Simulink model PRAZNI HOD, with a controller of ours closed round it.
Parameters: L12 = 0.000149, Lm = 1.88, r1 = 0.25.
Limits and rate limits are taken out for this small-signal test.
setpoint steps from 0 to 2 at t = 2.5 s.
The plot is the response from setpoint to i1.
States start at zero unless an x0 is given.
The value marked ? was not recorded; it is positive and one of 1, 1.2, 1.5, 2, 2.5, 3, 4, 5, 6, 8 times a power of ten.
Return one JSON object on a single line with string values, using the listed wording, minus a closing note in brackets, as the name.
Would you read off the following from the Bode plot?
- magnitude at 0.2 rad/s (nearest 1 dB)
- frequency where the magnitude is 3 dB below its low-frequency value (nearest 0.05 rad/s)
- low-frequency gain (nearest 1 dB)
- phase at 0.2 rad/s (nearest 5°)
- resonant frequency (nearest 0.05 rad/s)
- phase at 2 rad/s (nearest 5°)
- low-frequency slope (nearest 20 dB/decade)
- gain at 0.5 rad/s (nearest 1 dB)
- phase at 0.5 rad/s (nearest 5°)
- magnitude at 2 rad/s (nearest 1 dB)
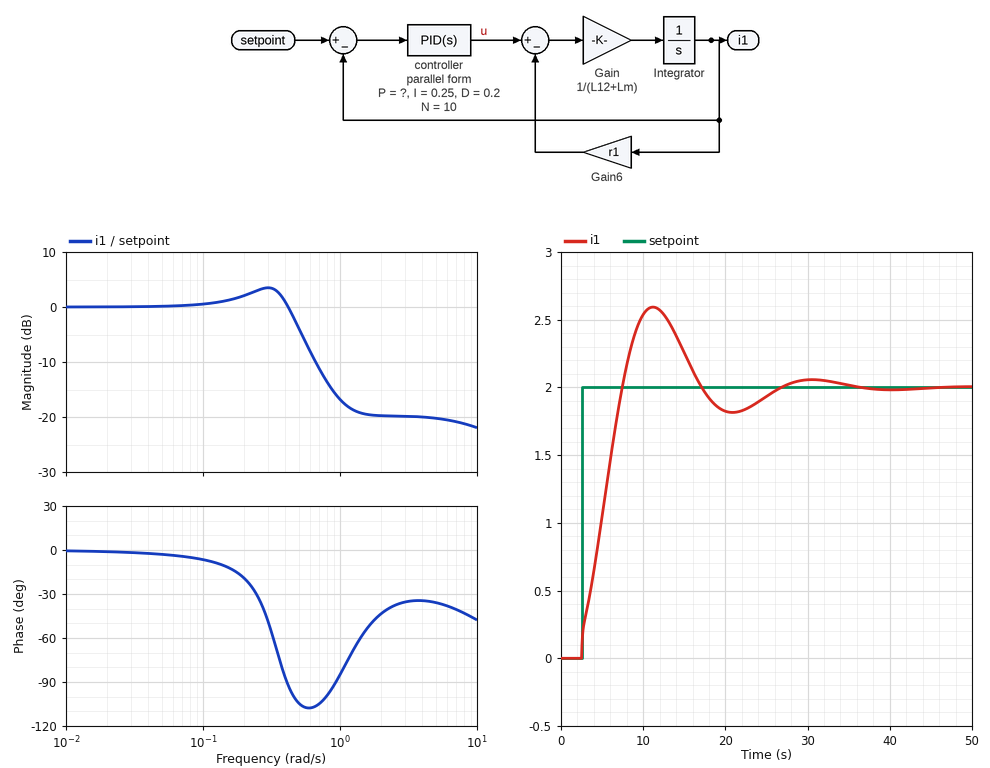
{"magnitude at 0.2 rad/s": "2 dB", "frequency where the magnitude is 3 dB below its low-frequency value": "0.50 rad/s", "low-frequency gain": "0 dB", "phase at 0.2 rad/s": "-20°", "resonant frequency": "0.30 rad/s", "phase at 2 rad/s": "-45°", "low-frequency slope": "0 dB/decade", "gain at 0.5 rad/s": "-4 dB", "phase at 0.5 rad/s": "-105°", "magnitude at 2 rad/s": "-20 dB"}
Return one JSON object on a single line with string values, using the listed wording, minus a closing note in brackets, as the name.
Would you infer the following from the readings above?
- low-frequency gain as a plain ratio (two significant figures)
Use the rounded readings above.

{"low-frequency gain as a plain ratio": "1.0"}
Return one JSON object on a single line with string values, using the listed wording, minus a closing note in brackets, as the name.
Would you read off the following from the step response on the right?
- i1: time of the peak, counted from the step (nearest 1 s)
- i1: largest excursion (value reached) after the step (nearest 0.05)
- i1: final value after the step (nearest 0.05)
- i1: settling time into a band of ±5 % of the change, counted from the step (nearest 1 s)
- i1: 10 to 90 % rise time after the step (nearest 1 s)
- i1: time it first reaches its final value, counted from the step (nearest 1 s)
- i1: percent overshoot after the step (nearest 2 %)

{"i1: time of the peak, counted from the step": "9 s", "i1: largest excursion (value reached) after the step": "2.60", "i1: final value after the step": "2.00", "i1: settling time into a band of ±5 % of the change, counted from the step": "22 s", "i1: 10 to 90 % rise time after the step": "4 s", "i1: time it first reaches its final value, counted from the step": "5 s", "i1: percent overshoot after the step": "30 %"}
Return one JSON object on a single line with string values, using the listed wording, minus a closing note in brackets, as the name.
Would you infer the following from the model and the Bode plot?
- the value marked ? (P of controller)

{"the value marked ?": "0.25"}
